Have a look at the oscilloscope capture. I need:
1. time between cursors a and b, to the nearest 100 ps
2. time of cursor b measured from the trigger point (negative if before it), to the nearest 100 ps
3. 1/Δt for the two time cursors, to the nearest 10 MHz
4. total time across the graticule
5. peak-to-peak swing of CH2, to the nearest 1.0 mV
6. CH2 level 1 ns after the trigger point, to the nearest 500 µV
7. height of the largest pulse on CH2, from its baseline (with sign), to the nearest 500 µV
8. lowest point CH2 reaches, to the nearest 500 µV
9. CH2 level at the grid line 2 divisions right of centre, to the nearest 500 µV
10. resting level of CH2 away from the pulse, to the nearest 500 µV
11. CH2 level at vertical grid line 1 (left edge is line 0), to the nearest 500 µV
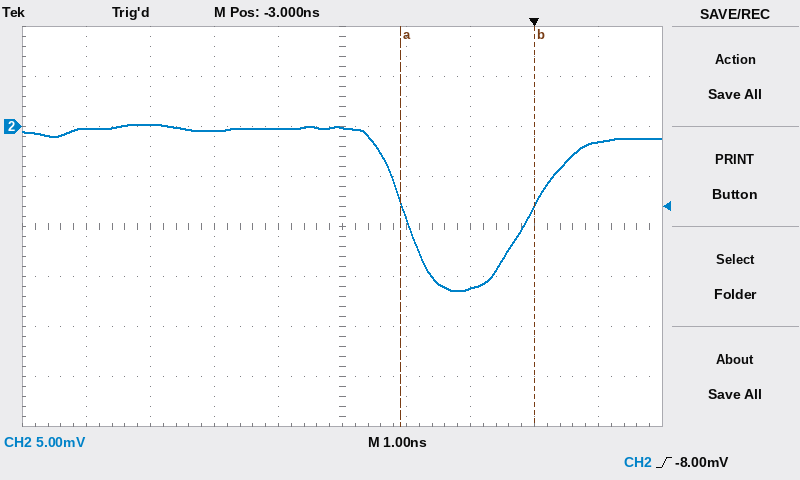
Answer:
2.1 ns
0.0 ns
480 MHz
10 ns
17.0 mV
-1.5 mV
-16.0 mV
-16.5 mV
-16.0 mV
-500 µV
0.0 mV
